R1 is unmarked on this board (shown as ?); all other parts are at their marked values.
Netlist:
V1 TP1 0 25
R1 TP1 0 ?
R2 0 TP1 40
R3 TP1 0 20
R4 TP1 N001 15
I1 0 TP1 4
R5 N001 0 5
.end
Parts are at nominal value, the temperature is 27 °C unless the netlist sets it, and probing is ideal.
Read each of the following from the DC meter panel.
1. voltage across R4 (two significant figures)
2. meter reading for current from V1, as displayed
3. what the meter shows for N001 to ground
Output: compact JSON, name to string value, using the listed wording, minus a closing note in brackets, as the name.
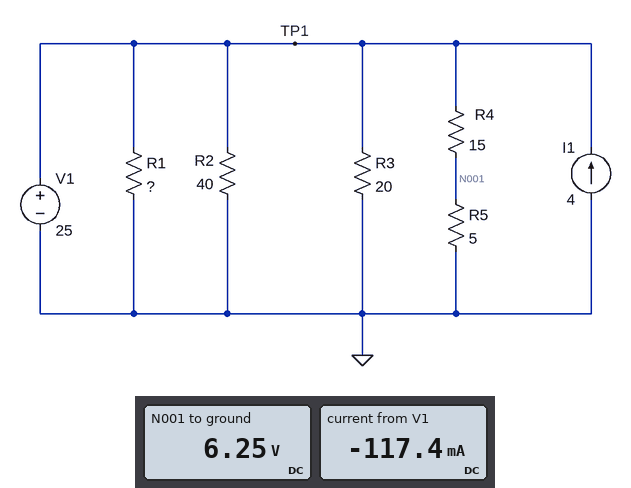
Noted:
{"voltage across R4": "19 V", "meter reading for current from V1, as displayed": "-117.4 mA", "what the meter shows for N001 to ground": "6.25 V"}
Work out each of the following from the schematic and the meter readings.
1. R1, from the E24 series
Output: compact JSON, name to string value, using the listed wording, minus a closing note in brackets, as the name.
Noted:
{"R1, from the E24 series": "33 Ω"}
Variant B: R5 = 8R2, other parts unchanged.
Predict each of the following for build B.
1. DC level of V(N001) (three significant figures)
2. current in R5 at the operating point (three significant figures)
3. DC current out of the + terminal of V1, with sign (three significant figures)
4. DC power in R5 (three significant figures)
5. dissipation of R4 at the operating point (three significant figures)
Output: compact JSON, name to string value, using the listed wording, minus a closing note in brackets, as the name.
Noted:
{"DC level of V(N001)": "8.84 V", "current in R5 at the operating point": "1.08 A", "DC current out of the + terminal of V1, with sign": "-290 mA", "DC power in R5": "9.52 W", "dissipation of R4 at the operating point": "17.4 W"}
